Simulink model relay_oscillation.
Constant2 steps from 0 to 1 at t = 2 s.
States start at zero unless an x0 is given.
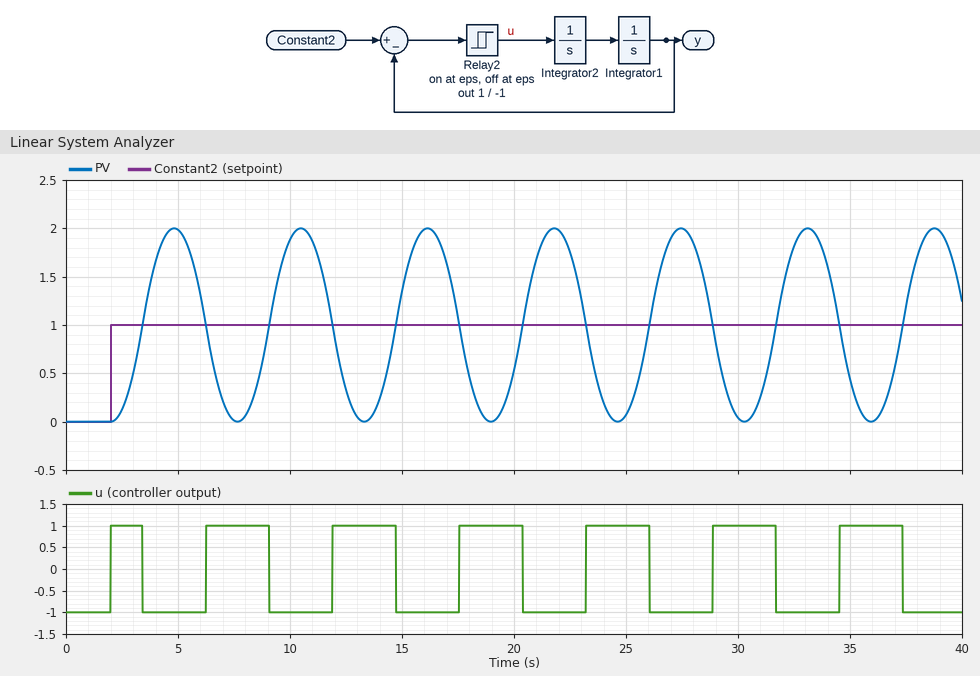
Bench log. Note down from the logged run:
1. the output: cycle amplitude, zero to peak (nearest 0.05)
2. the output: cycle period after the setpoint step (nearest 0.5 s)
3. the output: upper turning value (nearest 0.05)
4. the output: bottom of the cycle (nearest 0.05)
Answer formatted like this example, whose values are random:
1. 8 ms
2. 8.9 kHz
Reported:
1. 1.00
2. 5.5 s
3. 2.00
4. 0.00
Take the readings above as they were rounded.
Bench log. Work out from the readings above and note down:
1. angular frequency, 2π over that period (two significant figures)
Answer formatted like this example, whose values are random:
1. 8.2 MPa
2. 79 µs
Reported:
1. 1.1 rad/s
